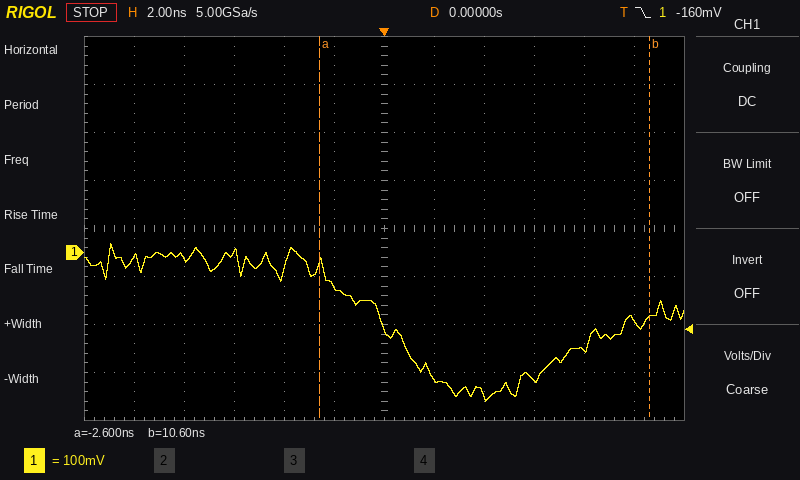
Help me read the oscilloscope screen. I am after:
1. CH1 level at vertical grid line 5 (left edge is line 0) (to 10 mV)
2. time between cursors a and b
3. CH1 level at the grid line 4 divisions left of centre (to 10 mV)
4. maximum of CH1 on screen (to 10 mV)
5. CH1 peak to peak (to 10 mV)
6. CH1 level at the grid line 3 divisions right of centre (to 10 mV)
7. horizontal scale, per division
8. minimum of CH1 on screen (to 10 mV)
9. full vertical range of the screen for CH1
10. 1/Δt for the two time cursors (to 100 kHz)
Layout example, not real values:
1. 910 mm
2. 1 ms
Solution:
1. -70 mV
2. 13.2 ns
3. -10 mV
4. 20 mV
5. 330 mV
6. -270 mV
7. 2 ns
8. -310 mV
9. 800 mV
10. 75.8 MHz
